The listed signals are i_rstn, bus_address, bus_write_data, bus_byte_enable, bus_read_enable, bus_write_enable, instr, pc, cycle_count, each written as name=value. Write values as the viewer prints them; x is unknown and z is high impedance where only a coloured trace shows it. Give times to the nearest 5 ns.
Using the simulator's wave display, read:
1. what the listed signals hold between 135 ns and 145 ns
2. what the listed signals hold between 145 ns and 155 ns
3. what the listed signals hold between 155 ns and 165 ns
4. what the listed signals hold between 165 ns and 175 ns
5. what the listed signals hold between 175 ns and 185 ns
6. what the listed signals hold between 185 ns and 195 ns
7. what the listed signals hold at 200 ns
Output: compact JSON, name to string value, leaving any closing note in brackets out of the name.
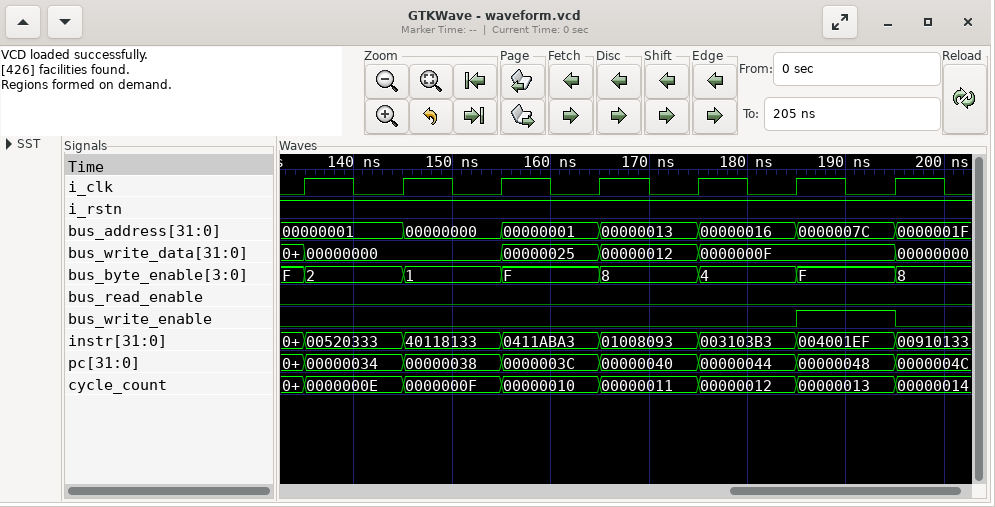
{"what the listed signals hold between 135 ns and 145 ns": "i_rstn=1, bus_address=00000001, bus_write_data=00000000, bus_byte_enable=2, bus_read_enable=0, bus_write_enable=0, instr=00520333, pc=00000034, cycle_count=0000000E", "what the listed signals hold between 145 ns and 155 ns": "i_rstn=1, bus_address=00000000, bus_write_data=00000000, bus_byte_enable=1, bus_read_enable=0, bus_write_enable=0, instr=40118133, pc=00000038, cycle_count=0000000F", "what the listed signals hold between 155 ns and 165 ns": "i_rstn=1, bus_address=00000001, bus_write_data=00000025, bus_byte_enable=F, bus_read_enable=0, bus_write_enable=0, instr=0411ABA3, pc=0000003C, cycle_count=00000010", "what the listed signals hold between 165 ns and 175 ns": "i_rstn=1, bus_address=00000013, bus_write_data=00000012, bus_byte_enable=8, bus_read_enable=0, bus_write_enable=0, instr=01008093, pc=00000040, cycle_count=00000011", "what the listed signals hold between 175 ns and 185 ns": "i_rstn=1, bus_address=00000016, bus_write_data=0000000F, bus_byte_enable=4, bus_read_enable=0, bus_write_enable=0, instr=003103B3, pc=00000044, cycle_count=00000012", "what the listed signals hold between 185 ns and 195 ns": "i_rstn=1, bus_address=0000007C, bus_write_data=0000000F, bus_byte_enable=F, bus_read_enable=0, bus_write_enable=1, instr=004001EF, pc=00000048, cycle_count=00000013", "what the listed signals hold at 200 ns": "i_rstn=1, bus_address=0000001F, bus_write_data=00000000, bus_byte_enable=8, bus_read_enable=0, bus_write_enable=0, instr=00910133, pc=0000004C, cycle_count=00000014"}
